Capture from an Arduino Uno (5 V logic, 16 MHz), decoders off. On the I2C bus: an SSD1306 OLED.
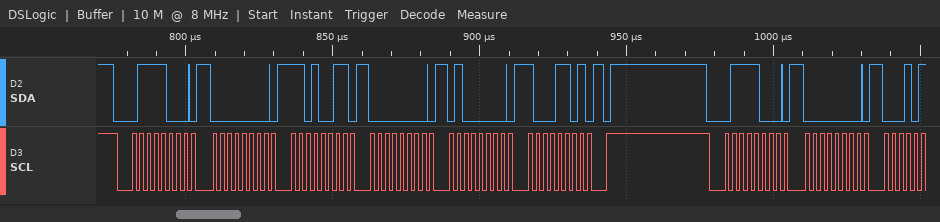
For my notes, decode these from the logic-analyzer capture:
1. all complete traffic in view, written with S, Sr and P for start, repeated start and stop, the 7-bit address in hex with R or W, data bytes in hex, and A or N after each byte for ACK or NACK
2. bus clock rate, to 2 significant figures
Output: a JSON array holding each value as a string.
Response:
["S 3CW A 00 A D3 A 00 A 40 A 8D A P S 3CW A 00 A", "400 kHz"]
